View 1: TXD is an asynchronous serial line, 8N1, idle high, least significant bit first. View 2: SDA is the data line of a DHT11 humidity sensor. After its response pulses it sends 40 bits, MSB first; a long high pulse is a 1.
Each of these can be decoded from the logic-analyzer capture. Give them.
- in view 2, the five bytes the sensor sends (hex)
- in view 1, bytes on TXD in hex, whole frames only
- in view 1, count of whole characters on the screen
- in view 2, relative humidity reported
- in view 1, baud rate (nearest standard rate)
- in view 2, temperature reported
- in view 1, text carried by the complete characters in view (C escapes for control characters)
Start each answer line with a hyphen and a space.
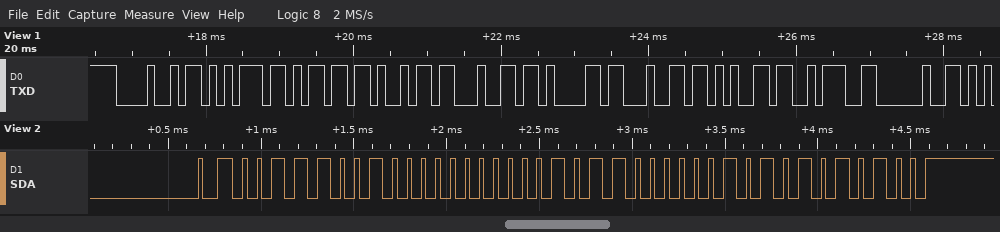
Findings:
- 39 00 16 05 54
- 0x48 0x75 0x6D 0x69 0x64 0x61 0x64 0x65 0x3A 0x20
- 10
- 57 %
- 9600 baud
- 22.5 °C
- "Humidade: "
